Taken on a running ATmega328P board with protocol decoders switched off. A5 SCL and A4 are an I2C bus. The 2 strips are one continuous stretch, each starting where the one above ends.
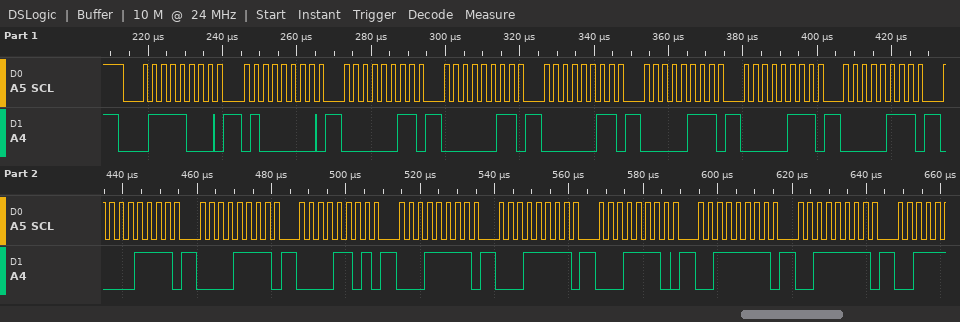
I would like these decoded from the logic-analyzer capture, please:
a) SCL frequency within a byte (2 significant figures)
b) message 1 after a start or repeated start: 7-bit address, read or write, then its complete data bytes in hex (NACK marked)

400 kHz
0x3C write: 40 03 03 03 07 07 07 0F 0F 0D 1F 1F 1E 3F 3F
